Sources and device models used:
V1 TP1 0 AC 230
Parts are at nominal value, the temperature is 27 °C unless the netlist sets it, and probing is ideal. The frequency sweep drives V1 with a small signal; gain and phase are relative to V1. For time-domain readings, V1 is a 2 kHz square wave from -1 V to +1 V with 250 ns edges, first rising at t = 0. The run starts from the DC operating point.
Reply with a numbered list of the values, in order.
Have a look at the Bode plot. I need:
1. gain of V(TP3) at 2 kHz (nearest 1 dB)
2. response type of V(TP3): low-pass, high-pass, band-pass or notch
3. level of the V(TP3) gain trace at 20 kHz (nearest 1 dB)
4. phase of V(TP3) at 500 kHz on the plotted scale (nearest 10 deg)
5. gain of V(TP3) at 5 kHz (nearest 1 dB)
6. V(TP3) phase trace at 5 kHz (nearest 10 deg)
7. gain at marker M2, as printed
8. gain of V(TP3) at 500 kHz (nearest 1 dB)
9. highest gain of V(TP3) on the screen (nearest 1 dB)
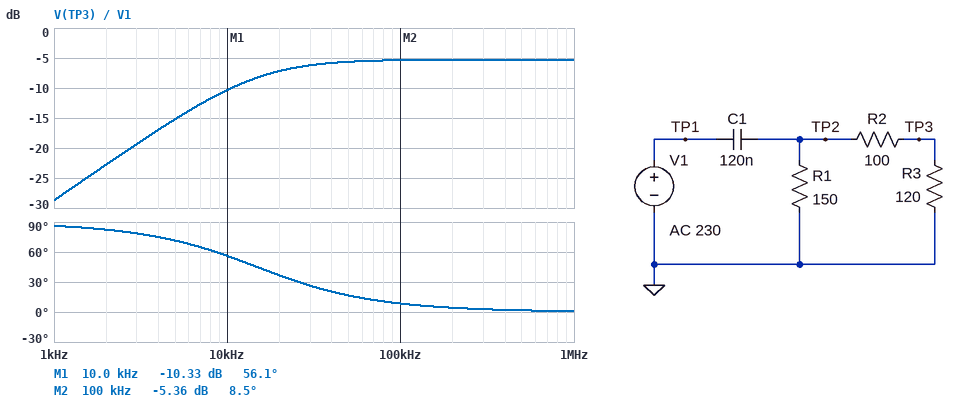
1. -23 dB
2. high-pass
3. -7 dB
4. 0 deg
5. -15 dB
6. 70 deg
7. -5.36 dB
8. -5 dB
9. -5 dB
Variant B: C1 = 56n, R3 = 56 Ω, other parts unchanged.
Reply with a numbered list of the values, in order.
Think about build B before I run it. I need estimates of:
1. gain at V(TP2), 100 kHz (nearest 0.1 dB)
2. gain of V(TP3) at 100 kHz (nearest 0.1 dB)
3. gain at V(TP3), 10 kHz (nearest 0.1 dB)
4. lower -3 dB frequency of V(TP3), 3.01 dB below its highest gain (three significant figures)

1. -0.6 dB
2. -9.5 dB
3. -20.6 dB
4. 37.2 kHz
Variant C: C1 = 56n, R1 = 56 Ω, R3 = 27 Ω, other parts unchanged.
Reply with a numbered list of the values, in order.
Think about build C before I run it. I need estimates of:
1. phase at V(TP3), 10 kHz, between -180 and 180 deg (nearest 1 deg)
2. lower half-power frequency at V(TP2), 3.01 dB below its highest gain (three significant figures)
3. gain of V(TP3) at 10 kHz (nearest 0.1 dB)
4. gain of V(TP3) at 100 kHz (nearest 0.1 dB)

1. 82 deg
2. 73.1 kHz
3. -30.8 dB
4. -15.3 dB
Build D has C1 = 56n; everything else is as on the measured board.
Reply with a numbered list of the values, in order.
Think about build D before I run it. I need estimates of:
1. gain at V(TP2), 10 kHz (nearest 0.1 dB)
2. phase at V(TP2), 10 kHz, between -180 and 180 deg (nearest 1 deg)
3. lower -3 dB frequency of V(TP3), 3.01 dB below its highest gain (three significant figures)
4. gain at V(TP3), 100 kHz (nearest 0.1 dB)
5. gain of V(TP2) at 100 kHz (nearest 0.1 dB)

1. -10.5 dB
2. 73 deg
3. 31.9 kHz
4. -5.7 dB
5. -0.4 dB
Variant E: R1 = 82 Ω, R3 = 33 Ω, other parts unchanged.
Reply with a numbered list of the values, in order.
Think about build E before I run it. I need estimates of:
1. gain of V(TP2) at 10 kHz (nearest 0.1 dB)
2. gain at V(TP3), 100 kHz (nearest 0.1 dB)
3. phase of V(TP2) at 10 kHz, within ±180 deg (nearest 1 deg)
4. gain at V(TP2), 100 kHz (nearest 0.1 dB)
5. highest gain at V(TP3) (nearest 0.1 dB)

1. -8.9 dB
2. -12.4 dB
3. 69 deg
4. -0.3 dB
5. -12.1 dB
